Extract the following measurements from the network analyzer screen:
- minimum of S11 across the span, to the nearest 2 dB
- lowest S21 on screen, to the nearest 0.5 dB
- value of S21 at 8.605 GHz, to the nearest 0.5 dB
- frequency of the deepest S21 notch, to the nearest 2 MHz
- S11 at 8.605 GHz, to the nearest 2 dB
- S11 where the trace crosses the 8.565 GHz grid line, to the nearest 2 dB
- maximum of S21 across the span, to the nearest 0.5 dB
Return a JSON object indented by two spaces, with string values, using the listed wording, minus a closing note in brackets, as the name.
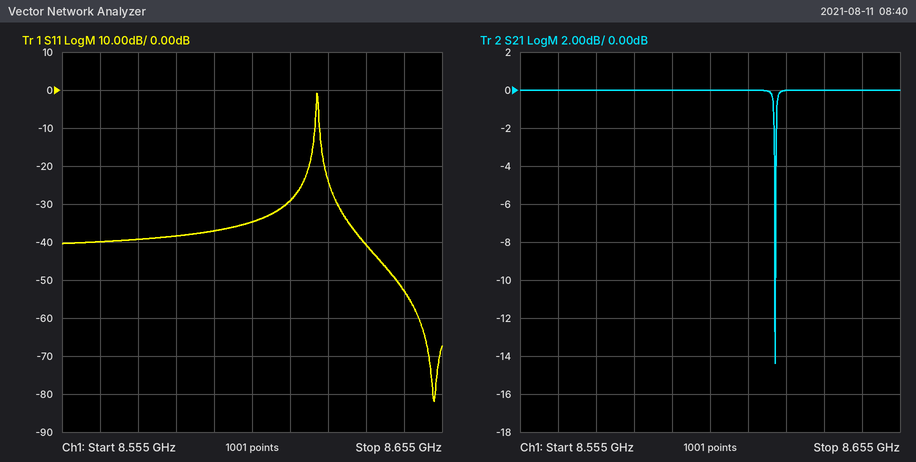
{
  "minimum of S11 across the span, to the nearest 2 dB": "-82 dB",
  "lowest S21 on screen, to the nearest 0.5 dB": "-14.5 dB",
  "value of S21 at 8.605 GHz, to the nearest 0.5 dB": "0.0 dB",
  "frequency of the deepest S21 notch, to the nearest 2 MHz": "8.622 GHz",
  "S11 at 8.605 GHz, to the nearest 2 dB": "-34 dB",
  "S11 where the trace crosses the 8.565 GHz grid line, to the nearest 2 dB": "-40 dB",
  "maximum of S21 across the span, to the nearest 0.5 dB": "0.0 dB"
}
